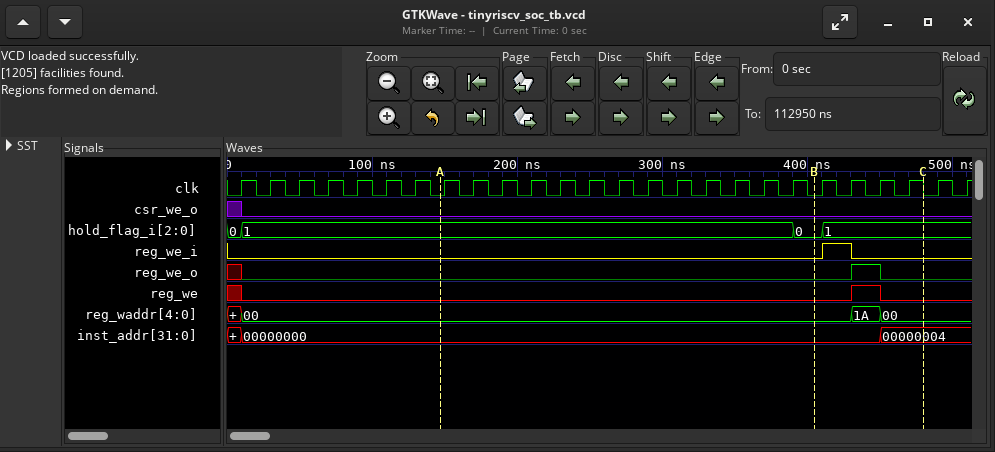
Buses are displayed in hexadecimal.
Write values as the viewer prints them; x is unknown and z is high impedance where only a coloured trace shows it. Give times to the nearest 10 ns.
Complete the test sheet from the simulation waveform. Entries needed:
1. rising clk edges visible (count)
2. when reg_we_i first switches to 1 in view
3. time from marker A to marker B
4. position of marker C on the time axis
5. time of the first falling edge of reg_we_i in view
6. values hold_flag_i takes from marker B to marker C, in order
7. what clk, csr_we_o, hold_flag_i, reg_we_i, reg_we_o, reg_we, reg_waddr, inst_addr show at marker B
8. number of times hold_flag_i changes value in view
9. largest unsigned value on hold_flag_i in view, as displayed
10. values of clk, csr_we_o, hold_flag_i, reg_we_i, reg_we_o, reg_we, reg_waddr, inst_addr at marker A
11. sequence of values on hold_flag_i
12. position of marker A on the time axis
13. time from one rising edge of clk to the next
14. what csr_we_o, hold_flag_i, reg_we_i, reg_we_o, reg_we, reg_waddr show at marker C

26
410 ns
260 ns
480 ns
430 ns
0, 1
clk=0, csr_we_o=0, hold_flag_i=0, reg_we_i=0, reg_we_o=0, reg_we=0, reg_waddr=00, inst_addr=00000000
3
1
clk=0, csr_we_o=0, hold_flag_i=1, reg_we_i=0, reg_we_o=0, reg_we=0, reg_waddr=00, inst_addr=00000000
0, 1, 0, 1
150 ns
20 ns
csr_we_o=0, hold_flag_i=1, reg_we_i=0, reg_we_o=0, reg_we=0, reg_waddr=00
